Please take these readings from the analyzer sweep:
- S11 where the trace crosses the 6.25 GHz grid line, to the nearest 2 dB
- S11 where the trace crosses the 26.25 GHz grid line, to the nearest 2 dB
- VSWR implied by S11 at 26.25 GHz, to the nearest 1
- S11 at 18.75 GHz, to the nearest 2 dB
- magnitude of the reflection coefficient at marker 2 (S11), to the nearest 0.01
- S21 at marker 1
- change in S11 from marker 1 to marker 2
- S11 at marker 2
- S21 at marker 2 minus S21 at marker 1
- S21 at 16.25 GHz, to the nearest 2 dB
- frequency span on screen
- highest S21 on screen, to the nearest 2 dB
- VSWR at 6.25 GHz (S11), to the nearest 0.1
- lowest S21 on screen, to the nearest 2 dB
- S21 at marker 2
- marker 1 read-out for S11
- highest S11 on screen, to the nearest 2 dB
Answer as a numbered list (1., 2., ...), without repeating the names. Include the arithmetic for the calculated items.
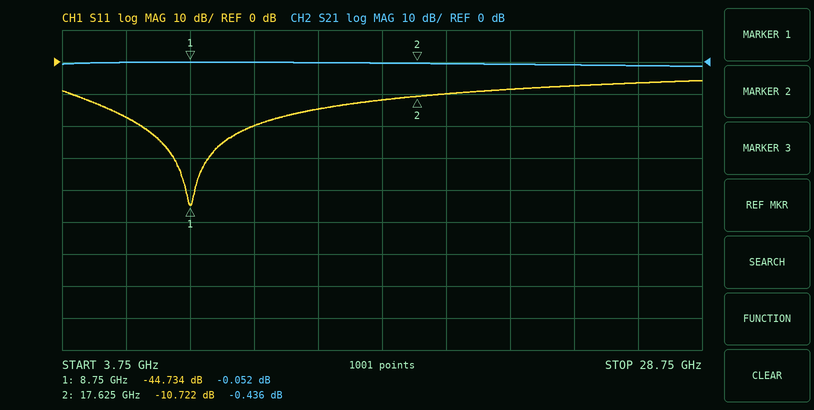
1. -18 dB
2. -6 dB
3. |Γ| = 10^(-6/20) = 0.5012; VSWR = (1 + 0.5012)/(1 − 0.5012) ≈ 3
4. -10 dB
5. 10^(-10.722/20) ≈ 0.29
6. -0.052 dB
7. -10.722 − (-44.734) = 34.012 dB
8. -10.722 dB
9. -0.436 − (-0.052) = -0.384 dB
10. 0 dB
11. 25 GHz
12. 0 dB
13. |Γ| = 10^(-18/20) = 0.1259; VSWR = (1 + 0.1259)/(1 − 0.1259) ≈ 1.3
14. -2 dB
15. -0.436 dB
16. -44.734 dB
17. -6 dB
